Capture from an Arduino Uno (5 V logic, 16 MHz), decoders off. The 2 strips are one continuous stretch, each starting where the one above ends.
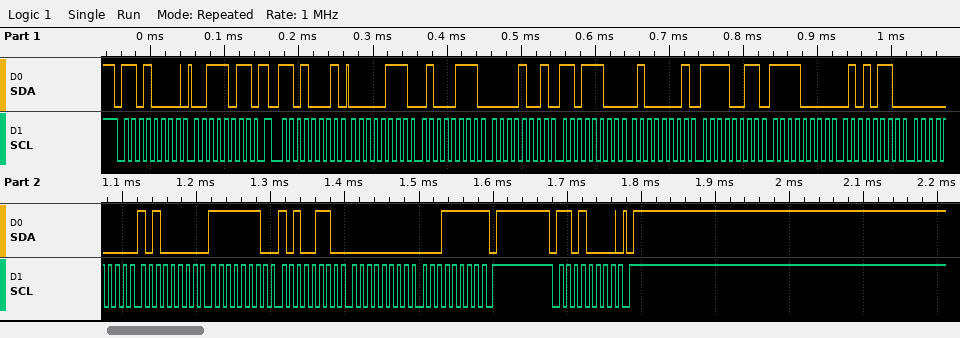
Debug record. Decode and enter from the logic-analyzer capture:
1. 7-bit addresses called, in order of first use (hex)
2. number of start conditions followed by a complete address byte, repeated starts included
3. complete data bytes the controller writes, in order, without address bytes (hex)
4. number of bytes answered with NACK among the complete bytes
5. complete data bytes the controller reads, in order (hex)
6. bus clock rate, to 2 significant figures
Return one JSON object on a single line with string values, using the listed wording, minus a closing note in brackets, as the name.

{"7-bit addresses called, in order of first use": "0x68", "number of start conditions followed by a complete address byte, repeated starts included": "3", "complete data bytes the controller writes, in order, without address bytes": "3B", "number of bytes answered with NACK among the complete bytes": "1", "complete data bytes the controller reads, in order": "07 47 09 DC 41 F3 F0 56 00 A0 FE A6 00 1F", "bus clock rate, to 2 significant figures": "100 kHz"}
